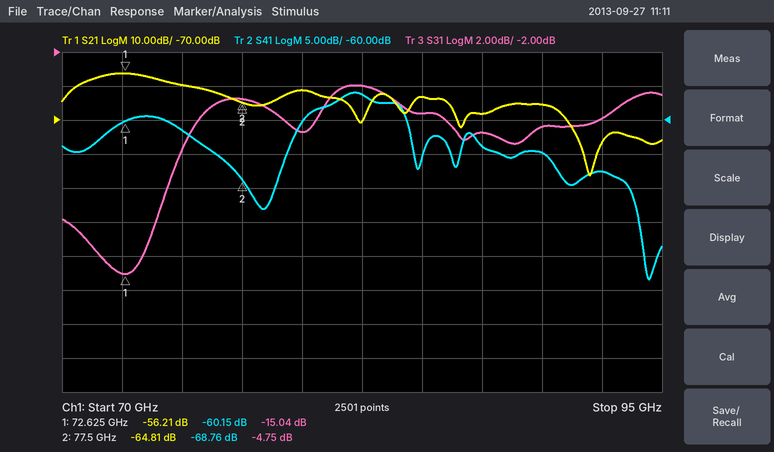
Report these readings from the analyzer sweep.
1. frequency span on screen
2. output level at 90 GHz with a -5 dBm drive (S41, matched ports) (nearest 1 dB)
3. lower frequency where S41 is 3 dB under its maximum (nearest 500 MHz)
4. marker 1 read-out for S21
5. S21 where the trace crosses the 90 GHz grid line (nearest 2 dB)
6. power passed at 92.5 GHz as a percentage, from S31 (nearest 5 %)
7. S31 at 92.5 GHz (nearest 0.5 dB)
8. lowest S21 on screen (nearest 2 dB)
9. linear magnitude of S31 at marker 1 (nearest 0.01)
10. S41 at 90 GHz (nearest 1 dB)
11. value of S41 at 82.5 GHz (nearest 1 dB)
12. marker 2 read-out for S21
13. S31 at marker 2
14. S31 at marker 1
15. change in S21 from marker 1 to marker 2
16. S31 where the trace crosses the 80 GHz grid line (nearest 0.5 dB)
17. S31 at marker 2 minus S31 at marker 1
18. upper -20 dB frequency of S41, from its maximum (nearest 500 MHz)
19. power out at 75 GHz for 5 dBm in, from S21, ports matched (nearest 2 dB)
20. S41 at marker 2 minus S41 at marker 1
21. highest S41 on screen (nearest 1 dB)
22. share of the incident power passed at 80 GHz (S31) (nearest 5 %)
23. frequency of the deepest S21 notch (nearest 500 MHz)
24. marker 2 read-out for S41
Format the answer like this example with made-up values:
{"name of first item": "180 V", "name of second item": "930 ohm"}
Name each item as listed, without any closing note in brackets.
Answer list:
{"frequency span on screen": "25 GHz", "output level at 90 GHz with a -5 dBm drive (S41, matched ports)": "-70 dBm", "lower frequency where S41 is 3 dB under its maximum": "80.5 GHz", "marker 1 read-out for S21": "-56.21 dB", "S21 where the trace crosses the 90 GHz grid line": "-66 dB", "power passed at 92.5 GHz as a percentage, from S31": "25 %", "S31 at 92.5 GHz": "-6.0 dB", "lowest S21 on screen": "-86 dB", "linear magnitude of S31 at marker 1": "0.18", "S41 at 90 GHz": "-65 dB", "value of S41 at 82.5 GHz": "-56 dB", "marker 2 read-out for S21": "-64.81 dB", "S31 at marker 2": "-4.75 dB", "S31 at marker 1": "-15.04 dB", "change in S21 from marker 1 to marker 2": "-8.60 dB", "S31 where the trace crosses the 80 GHz grid line": "-6.5 dB", "S31 at marker 2 minus S31 at marker 1": "10.29 dB", "upper -20 dB frequency of S41, from its maximum": "94.0 GHz", "power out at 75 GHz for 5 dBm in, from S21, ports matched": "-54 dBm", "S41 at marker 2 minus S41 at marker 1": "-8.61 dB", "highest S41 on screen": "-56 dB", "share of the incident power passed at 80 GHz (S31)": "20 %", "frequency of the deepest S21 notch": "92.0 GHz", "marker 2 read-out for S41": "-68.76 dB"}
